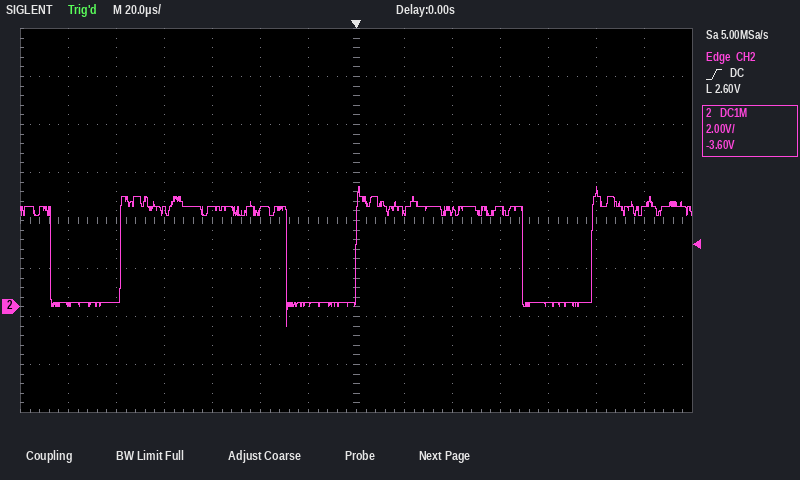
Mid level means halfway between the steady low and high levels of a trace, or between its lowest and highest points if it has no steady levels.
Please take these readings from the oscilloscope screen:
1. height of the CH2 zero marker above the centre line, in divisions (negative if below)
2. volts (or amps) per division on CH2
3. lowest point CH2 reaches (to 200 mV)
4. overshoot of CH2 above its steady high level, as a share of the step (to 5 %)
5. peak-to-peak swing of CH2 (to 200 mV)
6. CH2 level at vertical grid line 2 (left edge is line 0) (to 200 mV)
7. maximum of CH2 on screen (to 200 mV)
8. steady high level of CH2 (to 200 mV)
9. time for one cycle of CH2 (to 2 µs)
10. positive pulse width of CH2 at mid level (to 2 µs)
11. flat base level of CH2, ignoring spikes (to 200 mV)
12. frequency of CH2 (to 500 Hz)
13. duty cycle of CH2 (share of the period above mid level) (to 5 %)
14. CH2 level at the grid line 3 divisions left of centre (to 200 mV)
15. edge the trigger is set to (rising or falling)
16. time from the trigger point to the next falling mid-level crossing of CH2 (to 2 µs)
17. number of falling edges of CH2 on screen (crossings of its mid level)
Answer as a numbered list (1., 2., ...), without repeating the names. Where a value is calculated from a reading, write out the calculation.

1. -1.8 div
2. 2 V
3. -800 mV
4. 20 %
5. 5.0 V − (-800 mV) = 5.8 V
6. 200 mV
7. 5.0 V
8. 4.2 V
9. 98 µs
10. 70 µs
11. 200 mV
12. 1 / 98 µs ≈ 10.2 kHz, so 10.0 kHz to the nearest 500 Hz
13. 70 µs / 98 µs ≈ 71.4 %, so 70 % to the nearest 5 %
14. 4.2 V
15. rising
16. 70 µs
17. 3
